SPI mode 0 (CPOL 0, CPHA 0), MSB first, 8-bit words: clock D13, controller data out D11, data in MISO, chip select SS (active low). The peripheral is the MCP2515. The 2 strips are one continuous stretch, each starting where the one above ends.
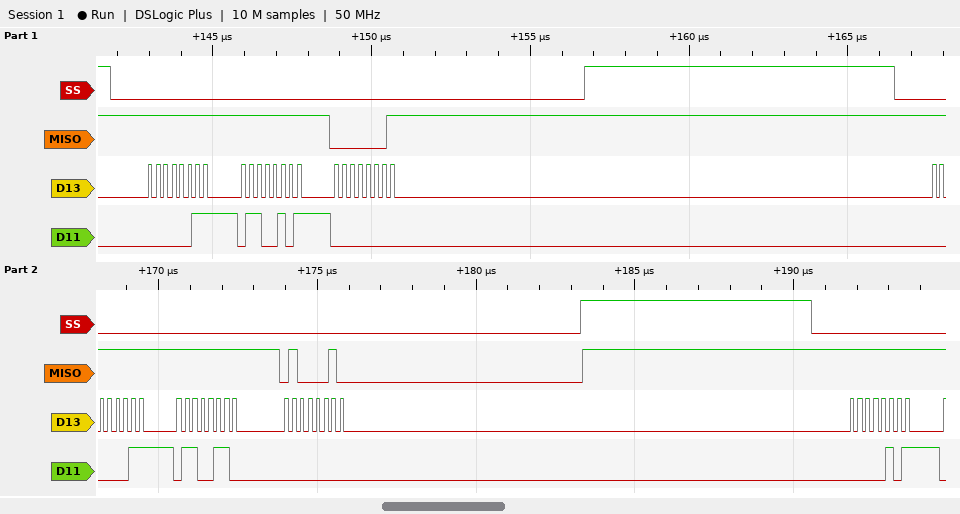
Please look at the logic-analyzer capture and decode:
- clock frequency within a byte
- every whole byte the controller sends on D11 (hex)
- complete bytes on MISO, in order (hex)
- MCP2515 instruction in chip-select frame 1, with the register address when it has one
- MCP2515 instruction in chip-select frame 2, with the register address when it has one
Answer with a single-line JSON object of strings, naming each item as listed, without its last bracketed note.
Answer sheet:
{"clock frequency within a byte": "4 MHz", "every whole byte the controller sends on D11": "03 65 00 03 66 00 05", "complete bytes on MISO, in order": "FF FF 01 FF FF 42 FF", "MCP2515 instruction in chip-select frame 1, with the register address when it has one": "READ 0x65", "MCP2515 instruction in chip-select frame 2, with the register address when it has one": "READ 0x66"}
